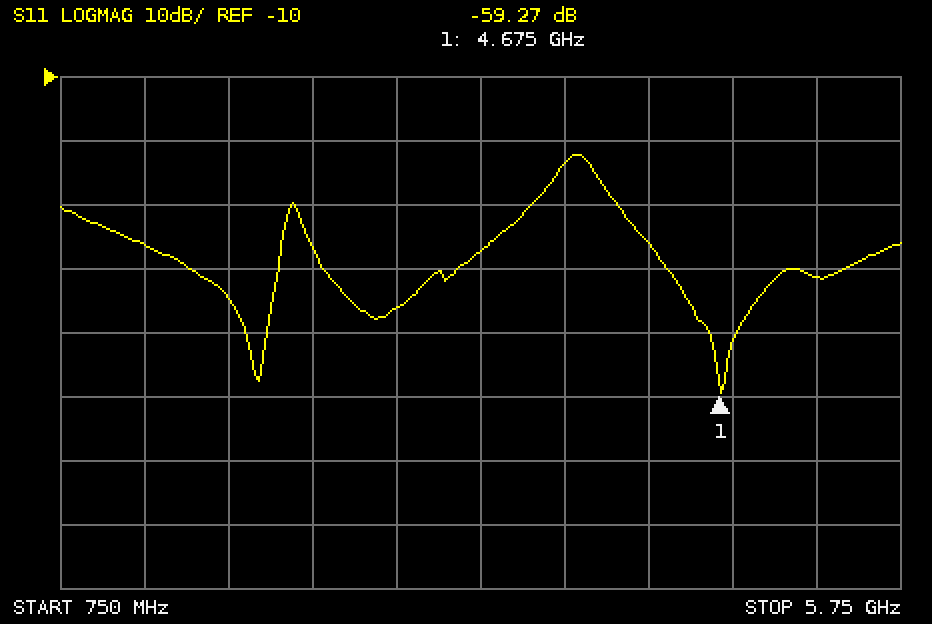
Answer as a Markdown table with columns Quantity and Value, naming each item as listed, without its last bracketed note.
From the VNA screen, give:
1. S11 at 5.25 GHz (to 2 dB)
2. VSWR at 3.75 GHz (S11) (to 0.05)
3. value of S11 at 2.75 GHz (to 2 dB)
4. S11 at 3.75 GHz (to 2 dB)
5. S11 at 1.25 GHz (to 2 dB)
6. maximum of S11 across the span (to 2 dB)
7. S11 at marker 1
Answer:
| Quantity | Value |
|---|---|
| S11 at 5.25 GHz | -42 dB |
| VSWR at 3.75 GHz (S11) | 1.15 |
| value of S11 at 2.75 GHz | -46 dB |
| S11 at 3.75 GHz | -24 dB |
| S11 at 1.25 GHz | -36 dB |
| maximum of S11 across the span | -22 dB |
| S11 at marker 1 | -59.27 dB |
